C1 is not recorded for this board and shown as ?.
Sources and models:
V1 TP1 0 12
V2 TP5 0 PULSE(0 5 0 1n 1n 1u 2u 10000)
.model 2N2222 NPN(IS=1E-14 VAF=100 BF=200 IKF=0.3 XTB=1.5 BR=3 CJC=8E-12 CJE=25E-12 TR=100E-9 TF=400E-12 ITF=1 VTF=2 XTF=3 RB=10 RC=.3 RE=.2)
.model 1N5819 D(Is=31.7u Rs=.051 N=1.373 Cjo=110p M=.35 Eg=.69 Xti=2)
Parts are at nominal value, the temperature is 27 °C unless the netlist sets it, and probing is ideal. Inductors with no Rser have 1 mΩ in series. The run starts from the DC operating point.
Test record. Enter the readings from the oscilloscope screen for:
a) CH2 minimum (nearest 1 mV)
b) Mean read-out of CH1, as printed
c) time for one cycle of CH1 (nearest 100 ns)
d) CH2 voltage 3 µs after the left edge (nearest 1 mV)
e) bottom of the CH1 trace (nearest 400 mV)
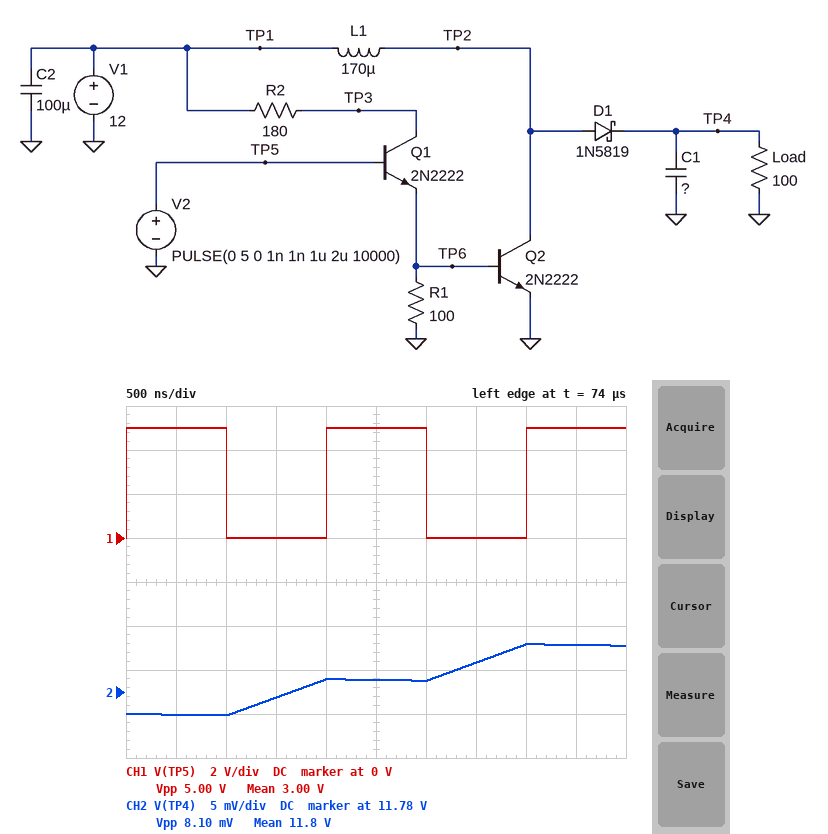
11.772 V
3.00 V
2.0 µs
11.776 V
0 V
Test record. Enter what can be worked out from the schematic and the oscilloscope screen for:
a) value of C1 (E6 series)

680 µF
